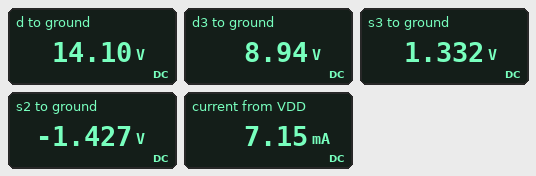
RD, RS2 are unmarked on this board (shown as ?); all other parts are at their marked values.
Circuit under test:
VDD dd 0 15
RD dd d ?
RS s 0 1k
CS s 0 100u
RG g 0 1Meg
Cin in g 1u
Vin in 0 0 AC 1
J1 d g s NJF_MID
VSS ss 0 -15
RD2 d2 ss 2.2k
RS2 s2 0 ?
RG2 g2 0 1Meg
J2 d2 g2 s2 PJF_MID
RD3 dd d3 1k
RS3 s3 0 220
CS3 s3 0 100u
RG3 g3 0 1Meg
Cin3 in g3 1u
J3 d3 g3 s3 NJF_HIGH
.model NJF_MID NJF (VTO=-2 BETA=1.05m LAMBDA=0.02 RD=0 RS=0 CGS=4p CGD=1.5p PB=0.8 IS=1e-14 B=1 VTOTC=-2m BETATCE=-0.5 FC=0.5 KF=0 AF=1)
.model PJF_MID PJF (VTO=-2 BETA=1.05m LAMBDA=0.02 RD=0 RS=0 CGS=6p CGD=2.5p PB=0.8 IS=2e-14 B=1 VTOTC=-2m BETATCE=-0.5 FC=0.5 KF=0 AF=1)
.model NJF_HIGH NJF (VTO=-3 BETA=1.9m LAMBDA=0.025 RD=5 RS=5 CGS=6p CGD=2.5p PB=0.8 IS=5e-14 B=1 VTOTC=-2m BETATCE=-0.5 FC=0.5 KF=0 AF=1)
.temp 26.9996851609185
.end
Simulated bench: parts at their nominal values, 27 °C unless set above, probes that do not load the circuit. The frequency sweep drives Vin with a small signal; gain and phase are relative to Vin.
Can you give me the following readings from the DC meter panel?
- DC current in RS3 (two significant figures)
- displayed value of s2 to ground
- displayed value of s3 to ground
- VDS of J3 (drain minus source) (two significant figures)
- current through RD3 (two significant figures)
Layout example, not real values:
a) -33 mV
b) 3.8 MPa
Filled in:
a) 6.1 mA
b) -1.427 V
c) 1.332 V
d) 7.6 V
e) 6.1 mA
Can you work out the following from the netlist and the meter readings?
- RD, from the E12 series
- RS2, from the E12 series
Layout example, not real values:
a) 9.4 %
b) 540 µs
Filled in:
a) 820 Ω
b) 3.3 kΩ
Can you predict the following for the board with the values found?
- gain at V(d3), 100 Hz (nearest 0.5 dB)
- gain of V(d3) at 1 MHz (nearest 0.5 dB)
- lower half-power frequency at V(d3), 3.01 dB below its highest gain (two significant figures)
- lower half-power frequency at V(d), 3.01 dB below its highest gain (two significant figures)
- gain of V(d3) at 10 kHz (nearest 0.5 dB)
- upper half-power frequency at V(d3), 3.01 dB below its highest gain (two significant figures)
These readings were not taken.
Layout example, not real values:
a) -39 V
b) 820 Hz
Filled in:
a) 16.0 dB
b) 16.0 dB
c) 14 Hz
d) 4.9 Hz
e) 16.0 dB
f) 260 MHz
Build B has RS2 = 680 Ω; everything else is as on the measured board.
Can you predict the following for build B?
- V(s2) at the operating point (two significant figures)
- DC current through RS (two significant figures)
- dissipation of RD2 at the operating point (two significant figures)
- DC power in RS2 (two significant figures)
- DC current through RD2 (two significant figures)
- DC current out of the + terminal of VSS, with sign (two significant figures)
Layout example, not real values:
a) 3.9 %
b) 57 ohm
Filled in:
a) -950 mV
b) 1.1 mA
c) 4.3 mW
d) 1.3 mW
e) 1.4 mA
f) -1.4 mA
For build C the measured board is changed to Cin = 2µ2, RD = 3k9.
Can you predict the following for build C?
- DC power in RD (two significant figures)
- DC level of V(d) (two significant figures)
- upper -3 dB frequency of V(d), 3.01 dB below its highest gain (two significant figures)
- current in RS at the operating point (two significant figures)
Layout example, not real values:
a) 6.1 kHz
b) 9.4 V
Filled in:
a) 4.5 mW
b) 11 V
c) 110 MHz
d) 1.1 mA
